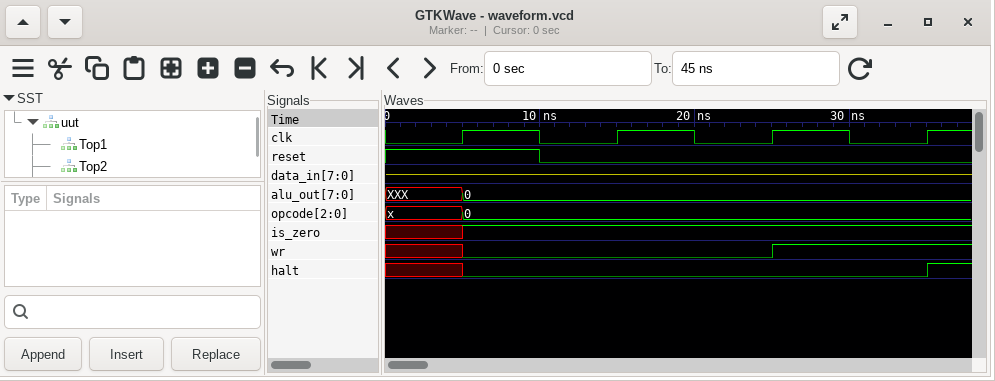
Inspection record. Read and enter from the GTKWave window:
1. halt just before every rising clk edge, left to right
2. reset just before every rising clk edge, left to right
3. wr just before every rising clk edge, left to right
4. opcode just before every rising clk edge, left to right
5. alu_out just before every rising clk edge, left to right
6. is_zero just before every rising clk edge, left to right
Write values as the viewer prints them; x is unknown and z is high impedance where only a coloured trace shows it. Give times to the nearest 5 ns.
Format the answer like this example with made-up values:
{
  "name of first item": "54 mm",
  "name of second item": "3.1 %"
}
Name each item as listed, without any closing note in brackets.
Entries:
{
  "halt just before every rising clk edge, left to right": "x 0 0 0",
  "reset just before every rising clk edge, left to right": "1 0 0 0",
  "wr just before every rising clk edge, left to right": "x 0 0 1",
  "opcode just before every rising clk edge, left to right": "x, 0, 0, 0",
  "alu_out just before every rising clk edge, left to right": "XXX, 0, 0, 0",
  "is_zero just before every rising clk edge, left to right": "x 1 1 1"
}
